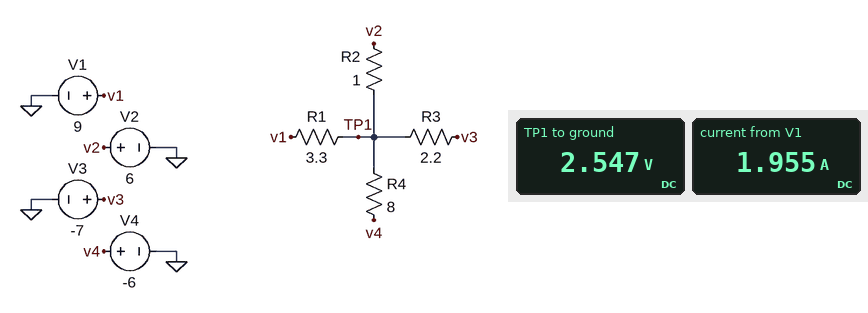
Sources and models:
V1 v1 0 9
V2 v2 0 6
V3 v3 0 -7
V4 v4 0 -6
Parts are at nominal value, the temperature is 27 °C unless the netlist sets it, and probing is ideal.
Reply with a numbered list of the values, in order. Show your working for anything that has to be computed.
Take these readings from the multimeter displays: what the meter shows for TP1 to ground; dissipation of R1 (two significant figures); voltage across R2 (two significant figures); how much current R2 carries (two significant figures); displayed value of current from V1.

1. 2.547 V
2. (9 V - 2.547 V)^2 / 3.3 Ω = 13 W
3. 6 V - 2.547 V = 3.5 V
4. (6 V - 2.547 V) / 1 Ω = 3.5 A
5. 1.955 A
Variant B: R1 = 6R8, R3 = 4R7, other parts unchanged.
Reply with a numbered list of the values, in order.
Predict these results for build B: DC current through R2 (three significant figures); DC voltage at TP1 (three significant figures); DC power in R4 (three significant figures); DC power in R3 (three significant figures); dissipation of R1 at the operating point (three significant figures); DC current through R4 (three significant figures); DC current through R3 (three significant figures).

1. 2.58 A
2. 3.42 V
3. 11.1 W
4. 23.1 W
5. 4.57 W
6. 1.18 A
7. 2.22 A
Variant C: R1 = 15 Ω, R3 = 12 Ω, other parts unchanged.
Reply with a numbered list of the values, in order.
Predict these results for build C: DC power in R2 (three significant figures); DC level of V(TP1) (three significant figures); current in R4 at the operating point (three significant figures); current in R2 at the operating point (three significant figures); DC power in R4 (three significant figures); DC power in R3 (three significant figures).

1. 3.49 W
2. 4.13 V
3. 1.27 A
4. 1.87 A
5. 12.8 W
6. 10.3 W
